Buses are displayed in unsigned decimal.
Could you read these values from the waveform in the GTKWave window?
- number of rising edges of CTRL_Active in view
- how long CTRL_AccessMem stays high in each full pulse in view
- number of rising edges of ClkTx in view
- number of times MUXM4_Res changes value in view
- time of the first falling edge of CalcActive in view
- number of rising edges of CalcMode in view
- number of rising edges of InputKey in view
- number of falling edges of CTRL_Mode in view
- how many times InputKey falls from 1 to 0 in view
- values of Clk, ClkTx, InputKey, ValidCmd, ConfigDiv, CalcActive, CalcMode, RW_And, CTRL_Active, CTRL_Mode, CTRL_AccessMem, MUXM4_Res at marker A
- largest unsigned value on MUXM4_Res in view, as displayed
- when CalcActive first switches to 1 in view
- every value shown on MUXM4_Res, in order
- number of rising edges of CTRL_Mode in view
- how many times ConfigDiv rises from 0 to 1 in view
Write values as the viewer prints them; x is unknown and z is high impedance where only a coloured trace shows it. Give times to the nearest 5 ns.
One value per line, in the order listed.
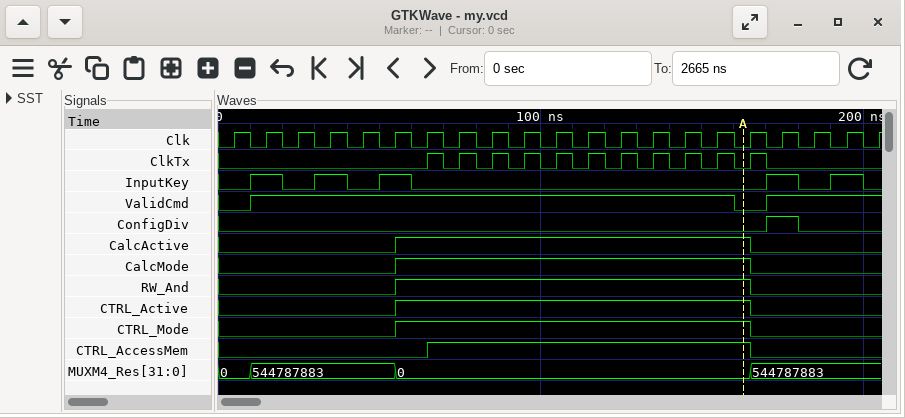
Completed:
1
100 ns
11
3
165 ns
1
5
1
5
Clk=0, ClkTx=0, InputKey=0, ValidCmd=0, ConfigDiv=0, CalcActive=1, CalcMode=1, RW_And=1, CTRL_Active=1, CTRL_Mode=1, CTRL_AccessMem=1, MUXM4_Res=0
544787883
55 ns
0, 544787883, 0, 544787883
1
1
